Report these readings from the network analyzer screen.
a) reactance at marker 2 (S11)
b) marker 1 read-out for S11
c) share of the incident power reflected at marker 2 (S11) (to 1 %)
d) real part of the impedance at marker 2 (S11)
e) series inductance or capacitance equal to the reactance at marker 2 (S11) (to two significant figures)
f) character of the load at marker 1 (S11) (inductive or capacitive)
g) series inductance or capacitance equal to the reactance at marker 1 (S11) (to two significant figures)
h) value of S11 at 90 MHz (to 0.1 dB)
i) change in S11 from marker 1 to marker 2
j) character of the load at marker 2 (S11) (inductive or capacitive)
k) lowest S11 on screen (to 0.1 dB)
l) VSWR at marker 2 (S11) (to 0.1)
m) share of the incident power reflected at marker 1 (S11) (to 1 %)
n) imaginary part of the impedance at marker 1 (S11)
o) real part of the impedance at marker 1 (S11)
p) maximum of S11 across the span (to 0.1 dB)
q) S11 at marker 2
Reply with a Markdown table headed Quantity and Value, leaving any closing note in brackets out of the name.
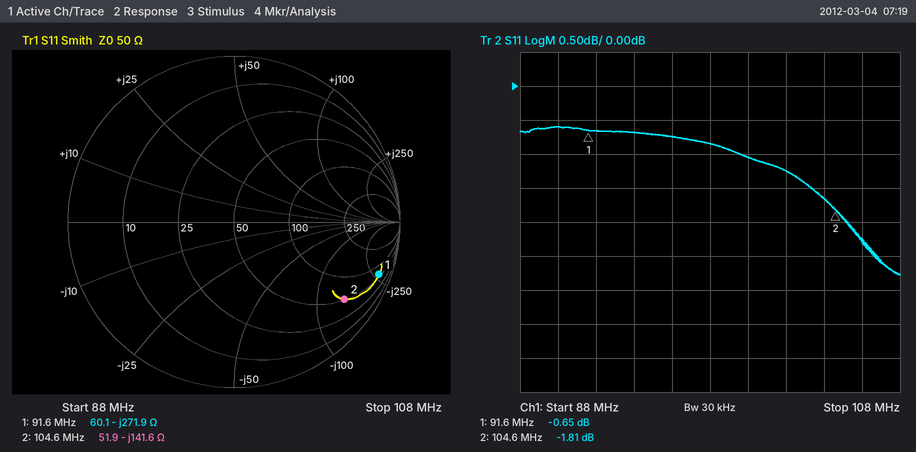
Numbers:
| Quantity | Value |
|---|---|
| reactance at marker 2 | -141.6 Ω |
| marker 1 read-out for S11 | -0.65 dB |
| share of the incident power reflected at marker 2 (S11) | 66 % |
| real part of the impedance at marker 2 | 51.9 Ω |
| series inductance or capacitance equal to the reactance at marker 2 (S11) | 11 pF |
| character of the load at marker 1 (S11) | capacitive |
| series inductance or capacitance equal to the reactance at marker 1 (S11) | 6.4 pF |
| value of S11 at 90 MHz | -0.6 dB |
| change in S11 from marker 1 to marker 2 | -1.16 dB |
| character of the load at marker 2 (S11) | capacitive |
| lowest S11 on screen | -2.8 dB |
| VSWR at marker 2 (S11) | 9.6 |
| share of the incident power reflected at marker 1 (S11) | 86 % |
| imaginary part of the impedance at marker 1 | -271.9 Ω |
| real part of the impedance at marker 1 | 60.1 Ω |
| maximum of S11 across the span | -0.6 dB |
| S11 at marker 2 | -1.81 dB |
